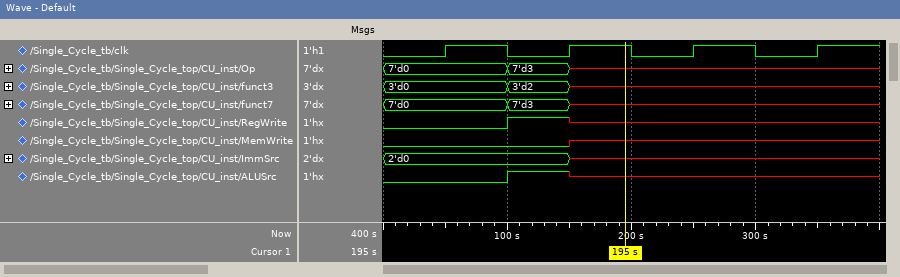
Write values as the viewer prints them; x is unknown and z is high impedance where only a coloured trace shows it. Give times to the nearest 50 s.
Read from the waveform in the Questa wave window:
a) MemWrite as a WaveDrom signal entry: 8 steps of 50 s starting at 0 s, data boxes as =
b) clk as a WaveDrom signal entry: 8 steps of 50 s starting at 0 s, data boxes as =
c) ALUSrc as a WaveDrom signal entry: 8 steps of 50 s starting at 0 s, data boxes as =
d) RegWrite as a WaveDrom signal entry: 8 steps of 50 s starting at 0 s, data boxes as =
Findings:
{name: 'MemWrite', wave: '0..x....'}
{name: 'clk', wave: '01010101'}
{name: 'ALUSrc', wave: '0.1x....'}
{name: 'RegWrite', wave: '0.1x....'}
